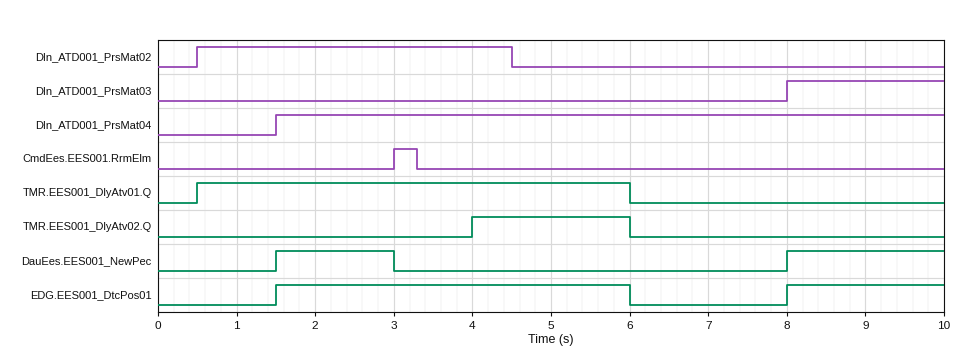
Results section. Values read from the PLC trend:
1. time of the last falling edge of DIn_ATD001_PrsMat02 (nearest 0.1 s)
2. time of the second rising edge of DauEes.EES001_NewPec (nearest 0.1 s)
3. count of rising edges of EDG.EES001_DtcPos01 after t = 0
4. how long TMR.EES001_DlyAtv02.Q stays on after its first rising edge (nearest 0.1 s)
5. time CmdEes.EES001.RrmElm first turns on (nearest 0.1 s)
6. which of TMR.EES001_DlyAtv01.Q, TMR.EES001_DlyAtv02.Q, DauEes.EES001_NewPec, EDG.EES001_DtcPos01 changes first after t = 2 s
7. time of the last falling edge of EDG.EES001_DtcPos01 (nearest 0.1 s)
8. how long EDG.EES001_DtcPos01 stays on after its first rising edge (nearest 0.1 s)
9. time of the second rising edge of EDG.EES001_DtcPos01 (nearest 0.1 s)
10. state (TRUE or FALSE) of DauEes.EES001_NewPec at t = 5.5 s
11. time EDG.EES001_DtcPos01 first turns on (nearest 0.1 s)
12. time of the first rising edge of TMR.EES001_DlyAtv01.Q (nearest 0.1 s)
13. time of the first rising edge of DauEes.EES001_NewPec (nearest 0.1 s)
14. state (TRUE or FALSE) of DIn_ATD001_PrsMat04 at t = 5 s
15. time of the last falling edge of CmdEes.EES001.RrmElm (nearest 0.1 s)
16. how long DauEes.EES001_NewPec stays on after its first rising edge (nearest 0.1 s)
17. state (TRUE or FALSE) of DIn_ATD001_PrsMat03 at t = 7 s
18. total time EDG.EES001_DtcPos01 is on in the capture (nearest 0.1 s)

4.5 s
8.0 s
2
2.0 s
3.0 s
DauEes.EES001_NewPec
6.0 s
4.5 s
8.0 s
FALSE
1.5 s
0.5 s
1.5 s
TRUE
3.3 s
1.5 s
FALSE
6.5 s
